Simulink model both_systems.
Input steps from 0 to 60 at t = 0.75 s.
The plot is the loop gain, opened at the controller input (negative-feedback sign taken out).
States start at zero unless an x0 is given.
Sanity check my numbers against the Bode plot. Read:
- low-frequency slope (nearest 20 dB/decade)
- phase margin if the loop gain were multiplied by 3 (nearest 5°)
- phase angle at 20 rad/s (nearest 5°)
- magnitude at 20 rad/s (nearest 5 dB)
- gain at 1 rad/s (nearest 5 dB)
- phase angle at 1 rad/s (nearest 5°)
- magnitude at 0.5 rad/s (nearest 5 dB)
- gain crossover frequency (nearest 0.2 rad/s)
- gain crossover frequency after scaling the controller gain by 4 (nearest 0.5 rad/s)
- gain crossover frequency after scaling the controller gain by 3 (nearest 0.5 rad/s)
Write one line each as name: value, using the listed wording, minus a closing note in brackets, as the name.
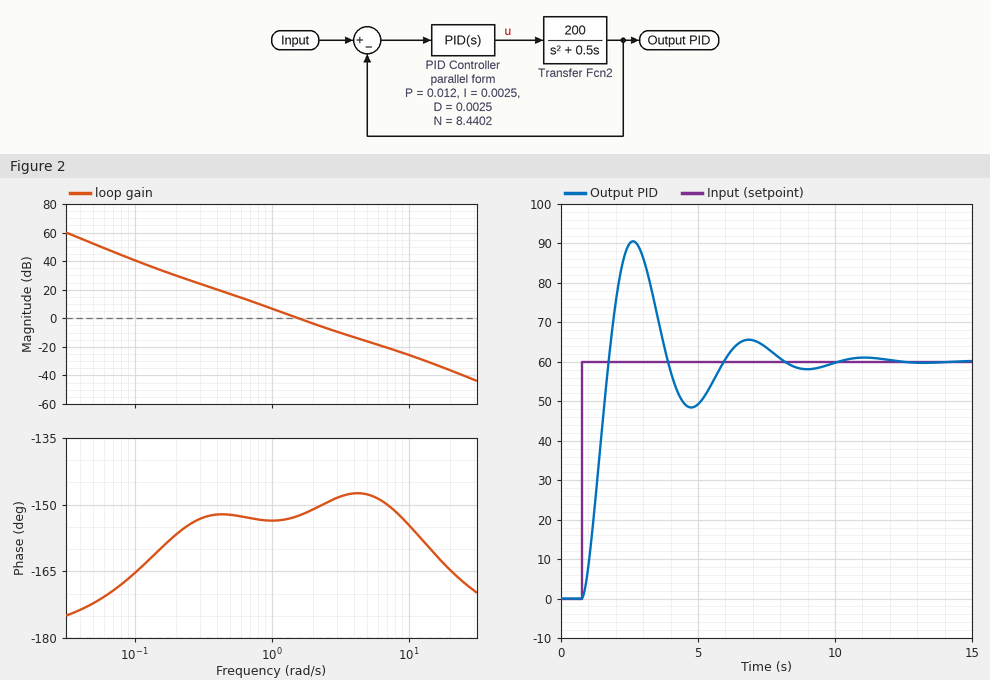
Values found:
low-frequency slope: -40 dB/decade
phase margin if the loop gain were multiplied by 3: 30°
phase angle at 20 rad/s: -165°
magnitude at 20 rad/s: -35 dB
gain at 1 rad/s: 5 dB
phase angle at 1 rad/s: -155°
magnitude at 0.5 rad/s: 15 dB
gain crossover frequency: 1.6 rad/s
gain crossover frequency after scaling the controller gain by 4: 3.5 rad/s
gain crossover frequency after scaling the controller gain by 3: 3.0 rad/s
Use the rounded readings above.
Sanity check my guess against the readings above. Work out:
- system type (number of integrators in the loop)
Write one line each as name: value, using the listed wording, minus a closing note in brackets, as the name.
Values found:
system type: 2
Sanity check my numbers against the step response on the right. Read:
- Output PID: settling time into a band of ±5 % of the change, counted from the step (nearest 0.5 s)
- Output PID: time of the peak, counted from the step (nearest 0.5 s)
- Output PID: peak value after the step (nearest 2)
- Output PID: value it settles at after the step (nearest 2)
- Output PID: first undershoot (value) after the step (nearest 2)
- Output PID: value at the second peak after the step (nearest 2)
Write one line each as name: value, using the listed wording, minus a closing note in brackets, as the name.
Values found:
Output PID: settling time into a band of ±5 % of the change, counted from the step: 7.0 s
Output PID: time of the peak, counted from the step: 2.0 s
Output PID: peak value after the step: 90
Output PID: value it settles at after the step: 60
Output PID: first undershoot (value) after the step: 48
Output PID: value at the second peak after the step: 66
